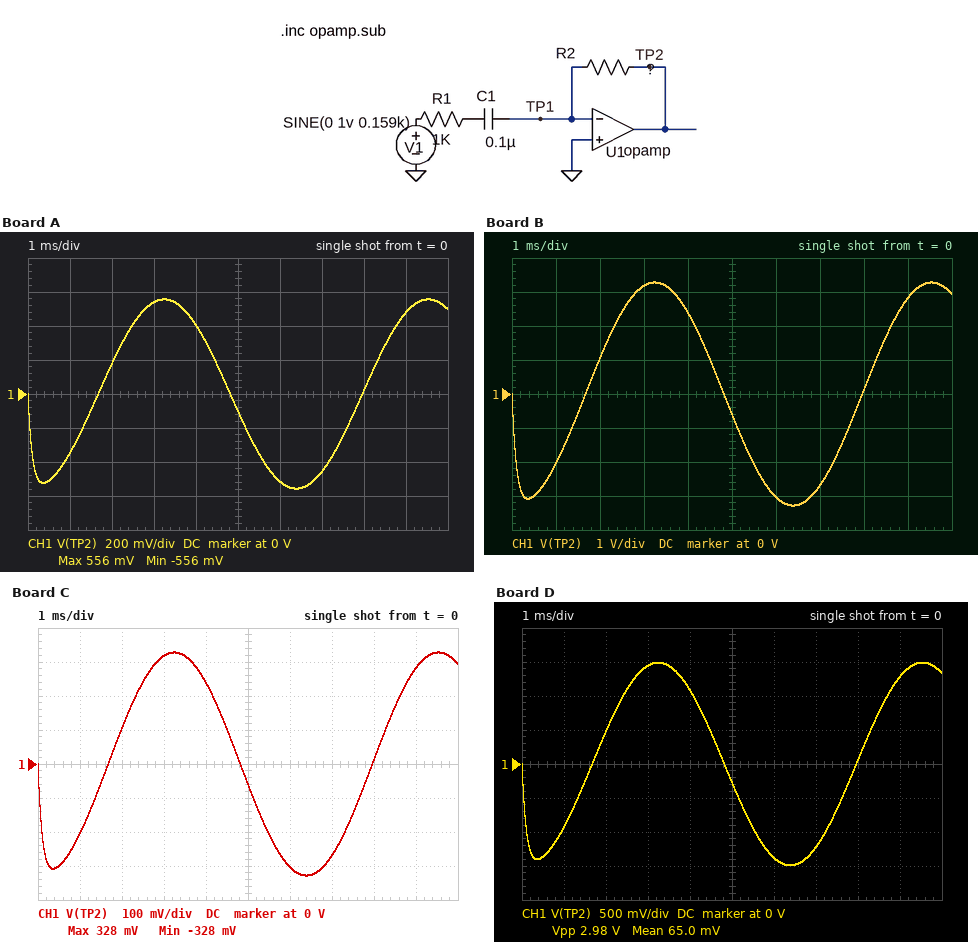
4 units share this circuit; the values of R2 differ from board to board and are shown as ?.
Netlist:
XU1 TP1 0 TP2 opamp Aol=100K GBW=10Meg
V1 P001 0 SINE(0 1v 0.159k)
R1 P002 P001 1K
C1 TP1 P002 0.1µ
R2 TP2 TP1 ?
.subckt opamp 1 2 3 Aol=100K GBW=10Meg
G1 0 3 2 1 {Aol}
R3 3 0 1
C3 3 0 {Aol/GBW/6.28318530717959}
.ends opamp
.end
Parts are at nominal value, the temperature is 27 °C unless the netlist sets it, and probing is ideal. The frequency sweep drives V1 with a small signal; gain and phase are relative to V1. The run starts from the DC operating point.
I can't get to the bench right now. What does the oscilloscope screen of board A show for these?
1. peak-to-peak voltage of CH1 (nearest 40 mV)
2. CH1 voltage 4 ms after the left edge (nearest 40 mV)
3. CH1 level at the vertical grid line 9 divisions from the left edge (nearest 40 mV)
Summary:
1.12 V
400 mV
480 mV
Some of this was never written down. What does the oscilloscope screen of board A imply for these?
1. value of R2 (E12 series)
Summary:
5.6 kΩ
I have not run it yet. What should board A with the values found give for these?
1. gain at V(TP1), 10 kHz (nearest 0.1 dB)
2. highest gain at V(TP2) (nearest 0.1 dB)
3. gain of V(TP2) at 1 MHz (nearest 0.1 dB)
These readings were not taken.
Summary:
-45.1 dB
15.0 dB
13.4 dB
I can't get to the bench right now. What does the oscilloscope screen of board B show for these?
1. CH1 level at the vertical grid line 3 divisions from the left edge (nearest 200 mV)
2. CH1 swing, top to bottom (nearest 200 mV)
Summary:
3.2 V
6.6 V
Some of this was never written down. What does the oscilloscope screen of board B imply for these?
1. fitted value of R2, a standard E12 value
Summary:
33 kΩ
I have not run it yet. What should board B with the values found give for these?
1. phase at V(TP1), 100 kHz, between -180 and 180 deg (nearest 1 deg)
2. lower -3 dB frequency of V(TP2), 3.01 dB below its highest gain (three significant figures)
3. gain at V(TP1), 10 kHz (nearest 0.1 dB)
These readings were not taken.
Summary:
72 deg
1.58 kHz
-29.7 dB
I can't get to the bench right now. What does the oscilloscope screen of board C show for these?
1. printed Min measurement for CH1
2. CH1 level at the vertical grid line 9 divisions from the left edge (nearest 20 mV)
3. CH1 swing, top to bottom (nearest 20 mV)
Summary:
-328 mV
280 mV
660 mV
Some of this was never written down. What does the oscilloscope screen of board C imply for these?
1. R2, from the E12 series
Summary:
3.3 kΩ
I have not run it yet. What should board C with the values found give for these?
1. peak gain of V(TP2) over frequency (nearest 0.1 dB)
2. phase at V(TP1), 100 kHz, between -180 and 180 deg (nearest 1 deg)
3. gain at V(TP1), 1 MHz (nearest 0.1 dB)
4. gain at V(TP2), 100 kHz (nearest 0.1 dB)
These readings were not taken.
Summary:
10.4 dB
88 deg
-10.4 dB
10.4 dB
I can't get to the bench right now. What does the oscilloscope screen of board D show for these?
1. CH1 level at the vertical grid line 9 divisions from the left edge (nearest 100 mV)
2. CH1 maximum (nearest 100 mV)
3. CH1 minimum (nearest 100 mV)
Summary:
1.3 V
1.5 V
-1.5 V
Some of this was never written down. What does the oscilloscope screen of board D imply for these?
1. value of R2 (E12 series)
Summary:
15 kΩ
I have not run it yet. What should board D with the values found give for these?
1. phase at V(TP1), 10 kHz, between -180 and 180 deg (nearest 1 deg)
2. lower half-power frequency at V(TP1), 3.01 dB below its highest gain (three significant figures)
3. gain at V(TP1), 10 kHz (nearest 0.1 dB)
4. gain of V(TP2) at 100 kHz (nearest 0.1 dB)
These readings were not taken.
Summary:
98 deg
624 kHz
-36.6 dB
23.4 dB
